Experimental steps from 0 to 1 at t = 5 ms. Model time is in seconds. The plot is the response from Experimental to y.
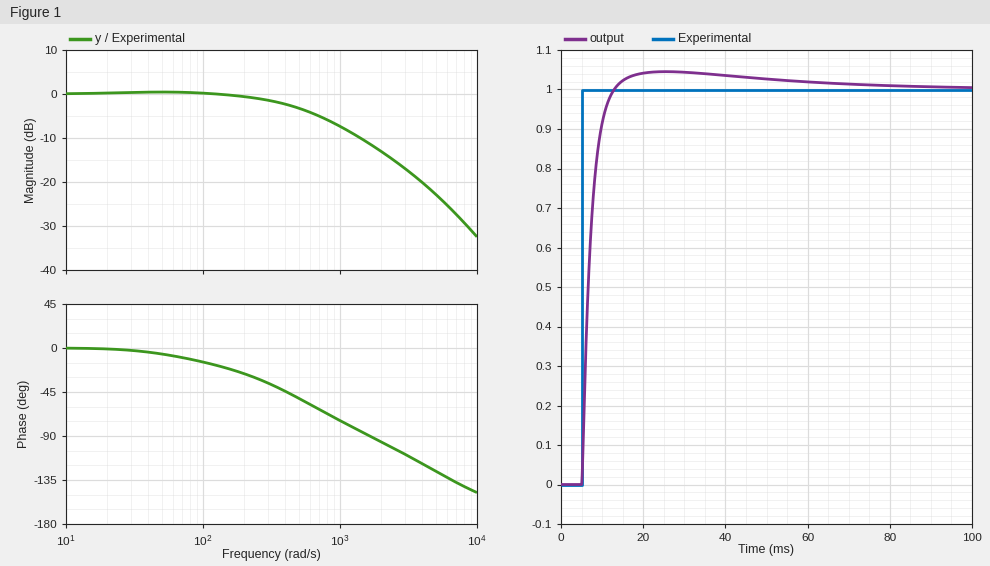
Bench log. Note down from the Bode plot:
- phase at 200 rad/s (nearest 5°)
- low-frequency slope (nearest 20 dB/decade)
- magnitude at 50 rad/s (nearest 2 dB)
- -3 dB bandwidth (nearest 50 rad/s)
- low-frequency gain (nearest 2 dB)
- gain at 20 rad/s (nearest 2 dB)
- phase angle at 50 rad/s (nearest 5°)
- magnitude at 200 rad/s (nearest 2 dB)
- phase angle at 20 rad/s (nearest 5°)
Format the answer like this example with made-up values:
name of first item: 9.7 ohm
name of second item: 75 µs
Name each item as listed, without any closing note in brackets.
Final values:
phase at 200 rad/s: -25°
low-frequency slope: 0 dB/decade
magnitude at 50 rad/s: 0 dB
-3 dB bandwidth: 450 rad/s
low-frequency gain: 0 dB
gain at 20 rad/s: 0 dB
phase angle at 50 rad/s: -5°
magnitude at 200 rad/s: 0 dB
phase angle at 20 rad/s: 0°
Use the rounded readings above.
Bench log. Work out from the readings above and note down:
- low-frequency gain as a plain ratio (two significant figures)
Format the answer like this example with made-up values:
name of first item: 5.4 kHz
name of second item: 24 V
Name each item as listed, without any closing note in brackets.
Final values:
low-frequency gain as a plain ratio: 1.0
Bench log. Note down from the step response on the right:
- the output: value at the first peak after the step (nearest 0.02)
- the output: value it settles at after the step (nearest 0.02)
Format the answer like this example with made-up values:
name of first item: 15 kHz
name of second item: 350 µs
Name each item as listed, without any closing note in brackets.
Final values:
the output: value at the first peak after the step: 1.04
the output: value it settles at after the step: 1.00
